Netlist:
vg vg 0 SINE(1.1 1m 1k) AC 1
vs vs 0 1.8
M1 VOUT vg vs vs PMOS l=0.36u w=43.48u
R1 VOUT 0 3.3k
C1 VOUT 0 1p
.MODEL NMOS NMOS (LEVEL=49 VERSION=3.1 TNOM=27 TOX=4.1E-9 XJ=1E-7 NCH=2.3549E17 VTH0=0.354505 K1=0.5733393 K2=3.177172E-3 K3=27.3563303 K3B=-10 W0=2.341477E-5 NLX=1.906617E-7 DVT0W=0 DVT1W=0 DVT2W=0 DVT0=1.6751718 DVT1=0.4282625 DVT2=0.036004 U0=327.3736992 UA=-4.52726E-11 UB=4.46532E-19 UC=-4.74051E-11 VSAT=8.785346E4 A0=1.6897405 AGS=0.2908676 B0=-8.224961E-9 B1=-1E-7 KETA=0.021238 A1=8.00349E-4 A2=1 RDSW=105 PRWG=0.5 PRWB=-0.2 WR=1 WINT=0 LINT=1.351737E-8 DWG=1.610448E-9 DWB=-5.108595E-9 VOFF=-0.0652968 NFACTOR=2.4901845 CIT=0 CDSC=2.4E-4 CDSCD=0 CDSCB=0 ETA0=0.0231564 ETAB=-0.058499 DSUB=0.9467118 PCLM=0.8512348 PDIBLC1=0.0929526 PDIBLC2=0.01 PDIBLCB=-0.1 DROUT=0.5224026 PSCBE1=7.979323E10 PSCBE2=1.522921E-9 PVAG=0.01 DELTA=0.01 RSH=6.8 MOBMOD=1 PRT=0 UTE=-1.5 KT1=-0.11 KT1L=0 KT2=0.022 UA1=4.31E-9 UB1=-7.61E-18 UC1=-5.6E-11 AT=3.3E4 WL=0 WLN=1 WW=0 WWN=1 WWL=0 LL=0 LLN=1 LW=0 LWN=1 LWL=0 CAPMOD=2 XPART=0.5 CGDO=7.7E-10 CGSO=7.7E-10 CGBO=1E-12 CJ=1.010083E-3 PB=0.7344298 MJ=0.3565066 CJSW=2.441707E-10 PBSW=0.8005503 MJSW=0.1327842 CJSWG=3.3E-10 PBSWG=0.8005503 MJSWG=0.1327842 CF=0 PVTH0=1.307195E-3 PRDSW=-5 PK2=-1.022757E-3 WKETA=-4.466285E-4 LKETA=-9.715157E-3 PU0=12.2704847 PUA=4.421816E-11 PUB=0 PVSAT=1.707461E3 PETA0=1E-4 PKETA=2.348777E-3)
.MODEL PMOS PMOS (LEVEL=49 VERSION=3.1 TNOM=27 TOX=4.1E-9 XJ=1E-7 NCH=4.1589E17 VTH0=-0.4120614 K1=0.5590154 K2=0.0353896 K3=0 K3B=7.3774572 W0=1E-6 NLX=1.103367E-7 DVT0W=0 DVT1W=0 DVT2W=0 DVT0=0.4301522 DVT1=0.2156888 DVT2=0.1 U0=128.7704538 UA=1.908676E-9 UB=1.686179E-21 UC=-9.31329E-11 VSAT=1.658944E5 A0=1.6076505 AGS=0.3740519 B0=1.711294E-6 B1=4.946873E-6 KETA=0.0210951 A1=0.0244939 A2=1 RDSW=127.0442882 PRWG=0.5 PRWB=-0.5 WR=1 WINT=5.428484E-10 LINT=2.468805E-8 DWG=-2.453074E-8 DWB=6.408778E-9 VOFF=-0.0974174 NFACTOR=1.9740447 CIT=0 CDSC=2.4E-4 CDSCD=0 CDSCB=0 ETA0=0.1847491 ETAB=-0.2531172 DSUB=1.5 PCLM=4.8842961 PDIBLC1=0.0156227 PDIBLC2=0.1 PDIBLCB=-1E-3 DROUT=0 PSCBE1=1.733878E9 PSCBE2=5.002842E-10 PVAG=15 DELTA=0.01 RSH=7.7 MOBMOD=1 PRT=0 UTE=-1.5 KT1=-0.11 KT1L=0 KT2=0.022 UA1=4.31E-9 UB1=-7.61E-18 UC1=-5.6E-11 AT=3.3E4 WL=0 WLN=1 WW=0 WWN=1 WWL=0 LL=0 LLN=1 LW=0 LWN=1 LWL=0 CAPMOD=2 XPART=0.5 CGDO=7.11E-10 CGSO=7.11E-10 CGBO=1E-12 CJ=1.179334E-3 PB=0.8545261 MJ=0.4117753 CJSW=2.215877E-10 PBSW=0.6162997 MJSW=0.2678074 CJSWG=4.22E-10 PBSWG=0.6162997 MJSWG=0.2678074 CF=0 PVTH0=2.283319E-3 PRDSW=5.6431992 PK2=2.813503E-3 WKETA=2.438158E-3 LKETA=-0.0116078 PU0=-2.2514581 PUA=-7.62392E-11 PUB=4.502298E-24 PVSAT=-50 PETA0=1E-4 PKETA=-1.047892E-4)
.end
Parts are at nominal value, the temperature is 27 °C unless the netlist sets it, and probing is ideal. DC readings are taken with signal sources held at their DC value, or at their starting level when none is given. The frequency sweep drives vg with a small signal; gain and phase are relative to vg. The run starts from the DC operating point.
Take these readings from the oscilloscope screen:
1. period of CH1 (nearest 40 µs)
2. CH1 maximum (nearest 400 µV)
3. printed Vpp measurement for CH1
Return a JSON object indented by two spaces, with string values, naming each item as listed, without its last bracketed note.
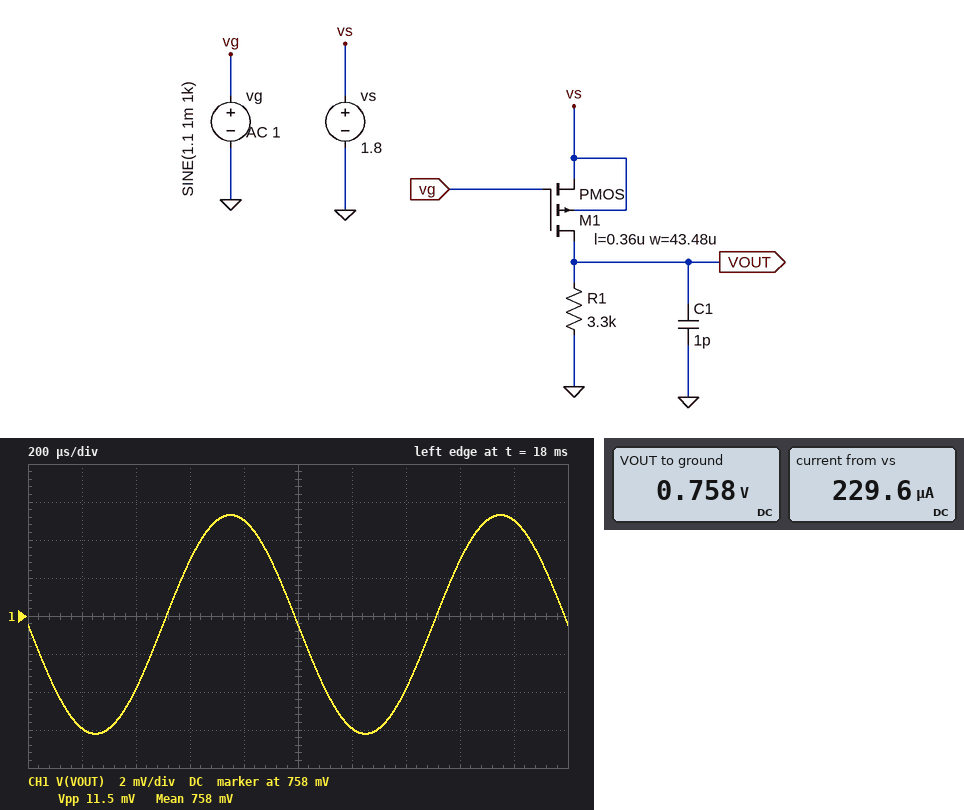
{
  "period of CH1": "1.00 ms",
  "CH1 maximum": "763.2 mV",
  "printed Vpp measurement for CH1": "11.5 mV"
}
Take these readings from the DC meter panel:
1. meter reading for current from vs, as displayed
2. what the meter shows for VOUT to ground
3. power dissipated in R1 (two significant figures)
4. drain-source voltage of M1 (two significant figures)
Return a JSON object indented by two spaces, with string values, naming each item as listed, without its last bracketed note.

{
  "meter reading for current from vs, as displayed": "229.6 µA",
  "what the meter shows for VOUT to ground": "0.758 V",
  "power dissipated in R1": "170 µW",
  "drain-source voltage of M1": "-1.0 V"
}
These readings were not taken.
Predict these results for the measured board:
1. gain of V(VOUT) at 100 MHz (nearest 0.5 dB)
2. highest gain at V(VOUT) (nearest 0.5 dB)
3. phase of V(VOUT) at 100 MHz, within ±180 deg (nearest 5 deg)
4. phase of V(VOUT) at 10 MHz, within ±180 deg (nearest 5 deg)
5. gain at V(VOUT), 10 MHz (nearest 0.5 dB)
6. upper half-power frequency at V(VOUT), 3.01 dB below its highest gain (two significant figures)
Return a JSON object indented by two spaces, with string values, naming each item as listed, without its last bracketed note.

{
  "gain of V(VOUT) at 100 MHz": "8.0 dB",
  "highest gain at V(VOUT)": "15.0 dB",
  "phase of V(VOUT) at 100 MHz, within ±180 deg": "115 deg",
  "phase of V(VOUT) at 10 MHz, within ±180 deg": "170 deg",
  "gain at V(VOUT), 10 MHz": "15.0 dB",
  "upper half-power frequency at V(VOUT), 3.01 dB below its highest gain": "49 MHz"
}
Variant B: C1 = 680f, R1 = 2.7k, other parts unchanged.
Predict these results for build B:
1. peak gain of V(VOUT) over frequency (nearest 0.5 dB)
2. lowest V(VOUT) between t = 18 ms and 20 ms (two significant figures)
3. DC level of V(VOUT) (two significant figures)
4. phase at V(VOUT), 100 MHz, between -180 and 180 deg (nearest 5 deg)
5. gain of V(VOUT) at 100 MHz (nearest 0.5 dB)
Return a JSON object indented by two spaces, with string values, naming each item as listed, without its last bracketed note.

{
  "peak gain of V(VOUT) over frequency": "13.5 dB",
  "lowest V(VOUT) between t = 18 ms and 20 ms": "620 mV",
  "DC level of V(VOUT)": "630 mV",
  "phase at V(VOUT), 100 MHz, between -180 and 180 deg": "130 deg",
  "gain of V(VOUT) at 100 MHz": "10.0 dB"
}
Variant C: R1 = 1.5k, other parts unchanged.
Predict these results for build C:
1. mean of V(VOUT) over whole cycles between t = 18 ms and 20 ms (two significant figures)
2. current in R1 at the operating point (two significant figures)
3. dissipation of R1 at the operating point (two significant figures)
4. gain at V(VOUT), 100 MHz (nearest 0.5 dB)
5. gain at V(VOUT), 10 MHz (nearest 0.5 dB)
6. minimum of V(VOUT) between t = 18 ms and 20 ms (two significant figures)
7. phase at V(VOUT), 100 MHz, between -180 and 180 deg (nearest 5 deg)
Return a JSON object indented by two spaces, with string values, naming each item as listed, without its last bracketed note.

{
  "mean of V(VOUT) over whole cycles between t = 18 ms and 20 ms": "360 mV",
  "current in R1 at the operating point": "240 µA",
  "dissipation of R1 at the operating point": "84 µW",
  "gain at V(VOUT), 100 MHz": "6.0 dB",
  "gain at V(VOUT), 10 MHz": "9.0 dB",
  "minimum of V(VOUT) between t = 18 ms and 20 ms": "350 mV",
  "phase at V(VOUT), 100 MHz, between -180 and 180 deg": "135 deg"
}
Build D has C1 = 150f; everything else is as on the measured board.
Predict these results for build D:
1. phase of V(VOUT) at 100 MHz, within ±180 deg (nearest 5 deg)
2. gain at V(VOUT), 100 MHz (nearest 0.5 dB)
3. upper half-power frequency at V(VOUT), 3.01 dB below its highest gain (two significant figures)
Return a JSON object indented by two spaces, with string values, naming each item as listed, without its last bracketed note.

{
  "phase of V(VOUT) at 100 MHz, within ±180 deg": "160 deg",
  "gain at V(VOUT), 100 MHz": "14.5 dB",
  "upper half-power frequency at V(VOUT), 3.01 dB below its highest gain": "260 MHz"
}
